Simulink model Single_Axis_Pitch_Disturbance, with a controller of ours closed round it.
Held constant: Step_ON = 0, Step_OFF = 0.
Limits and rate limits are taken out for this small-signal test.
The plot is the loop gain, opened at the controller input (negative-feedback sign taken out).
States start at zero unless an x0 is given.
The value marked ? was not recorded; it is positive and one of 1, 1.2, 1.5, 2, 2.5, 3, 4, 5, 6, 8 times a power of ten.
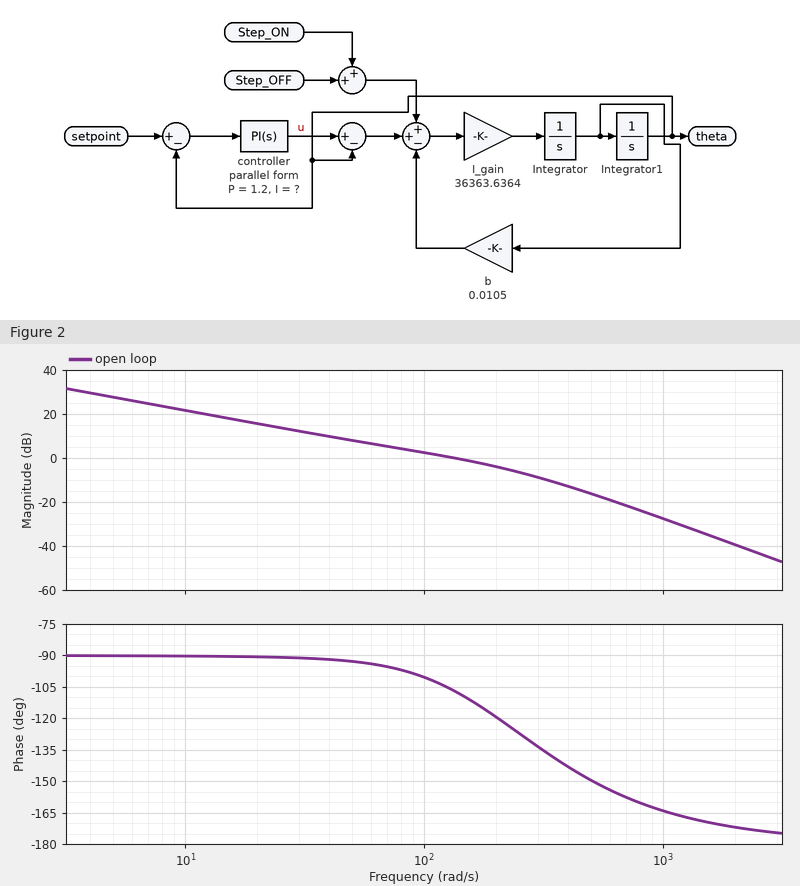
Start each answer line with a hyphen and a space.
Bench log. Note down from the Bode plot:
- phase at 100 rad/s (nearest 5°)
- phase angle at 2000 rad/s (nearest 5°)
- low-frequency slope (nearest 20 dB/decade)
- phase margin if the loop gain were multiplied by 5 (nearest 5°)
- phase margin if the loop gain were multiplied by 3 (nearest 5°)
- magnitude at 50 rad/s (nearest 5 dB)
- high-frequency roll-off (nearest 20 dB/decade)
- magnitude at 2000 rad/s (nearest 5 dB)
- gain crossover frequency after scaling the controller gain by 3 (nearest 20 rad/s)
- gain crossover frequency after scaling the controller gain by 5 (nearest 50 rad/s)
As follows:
- -100°
- -170°
- -20 dB/decade
- 35°
- 45°
- 10 dB
- -40 dB/decade
- -40 dB
- 320 rad/s
- 450 rad/s
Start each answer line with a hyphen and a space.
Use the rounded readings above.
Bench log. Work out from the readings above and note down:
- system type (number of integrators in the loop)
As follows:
- 1
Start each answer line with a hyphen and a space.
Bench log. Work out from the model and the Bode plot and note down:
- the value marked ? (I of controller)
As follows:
- 120
